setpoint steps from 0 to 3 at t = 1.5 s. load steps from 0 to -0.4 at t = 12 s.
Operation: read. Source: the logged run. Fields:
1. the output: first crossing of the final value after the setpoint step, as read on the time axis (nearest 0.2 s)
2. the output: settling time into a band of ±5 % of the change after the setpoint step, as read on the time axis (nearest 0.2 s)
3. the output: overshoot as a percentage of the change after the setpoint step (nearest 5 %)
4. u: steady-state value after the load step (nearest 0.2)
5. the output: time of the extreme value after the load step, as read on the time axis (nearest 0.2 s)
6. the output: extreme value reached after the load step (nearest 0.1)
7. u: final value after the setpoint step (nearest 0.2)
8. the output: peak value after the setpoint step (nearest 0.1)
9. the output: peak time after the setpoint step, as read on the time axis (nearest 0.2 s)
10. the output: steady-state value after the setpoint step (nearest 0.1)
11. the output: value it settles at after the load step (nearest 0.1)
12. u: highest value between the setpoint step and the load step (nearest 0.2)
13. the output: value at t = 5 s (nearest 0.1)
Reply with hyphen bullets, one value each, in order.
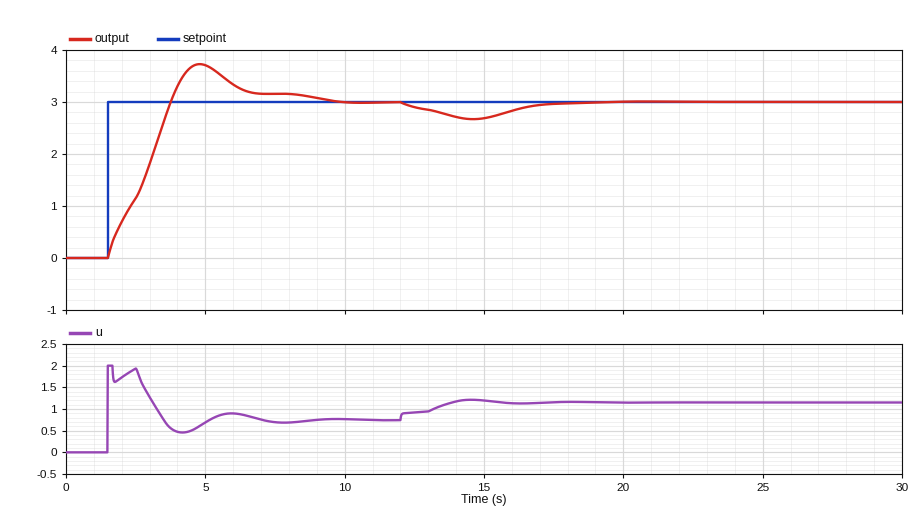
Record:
- 3.8 s
- 8.2 s
- 25 %
- 1.2
- 14.6 s
- 2.7
- 0.8
- 3.7
- 4.8 s
- 3.0
- 3.0
- 2.0
- 3.7
